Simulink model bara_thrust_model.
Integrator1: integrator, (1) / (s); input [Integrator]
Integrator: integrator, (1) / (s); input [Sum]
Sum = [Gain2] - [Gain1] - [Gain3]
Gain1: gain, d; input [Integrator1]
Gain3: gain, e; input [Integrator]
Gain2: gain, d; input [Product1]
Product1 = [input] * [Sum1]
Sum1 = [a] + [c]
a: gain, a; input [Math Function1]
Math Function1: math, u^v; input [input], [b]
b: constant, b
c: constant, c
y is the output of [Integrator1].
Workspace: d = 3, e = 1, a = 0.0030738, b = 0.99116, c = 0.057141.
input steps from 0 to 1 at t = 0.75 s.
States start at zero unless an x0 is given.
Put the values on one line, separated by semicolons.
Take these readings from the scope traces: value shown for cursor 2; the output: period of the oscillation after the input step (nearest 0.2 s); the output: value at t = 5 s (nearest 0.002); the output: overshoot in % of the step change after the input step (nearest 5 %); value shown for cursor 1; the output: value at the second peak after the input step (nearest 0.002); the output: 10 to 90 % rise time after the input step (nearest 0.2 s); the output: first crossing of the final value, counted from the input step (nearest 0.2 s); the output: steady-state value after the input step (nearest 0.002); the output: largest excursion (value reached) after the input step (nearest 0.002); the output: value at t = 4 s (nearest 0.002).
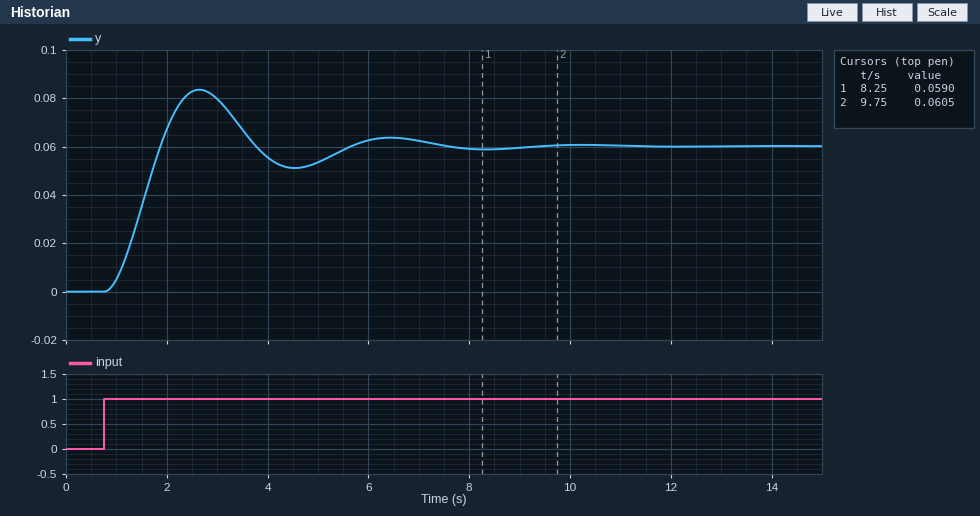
0.0605; 3.8 s; 0.054; 40 %; 0.0590; 0.064; 0.8 s; 1.2 s; 0.060; 0.084; 0.056
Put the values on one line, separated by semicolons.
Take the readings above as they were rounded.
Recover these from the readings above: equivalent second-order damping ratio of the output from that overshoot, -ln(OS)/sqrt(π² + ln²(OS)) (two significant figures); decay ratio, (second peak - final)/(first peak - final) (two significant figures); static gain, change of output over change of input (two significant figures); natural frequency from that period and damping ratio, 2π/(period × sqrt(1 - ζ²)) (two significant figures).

0.28; 0.17; 0.060; 1.7 rad/s
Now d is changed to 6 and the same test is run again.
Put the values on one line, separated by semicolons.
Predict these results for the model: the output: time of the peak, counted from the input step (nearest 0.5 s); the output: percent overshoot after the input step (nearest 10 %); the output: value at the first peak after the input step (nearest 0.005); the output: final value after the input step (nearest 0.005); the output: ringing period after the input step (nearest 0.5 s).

1.5 s; 50 %; 0.090; 0.060; 2.5 s
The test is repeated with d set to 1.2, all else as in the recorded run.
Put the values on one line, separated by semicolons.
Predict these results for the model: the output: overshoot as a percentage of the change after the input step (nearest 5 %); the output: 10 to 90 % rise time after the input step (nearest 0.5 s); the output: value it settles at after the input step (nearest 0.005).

20 %; 1.5 s; 0.060
